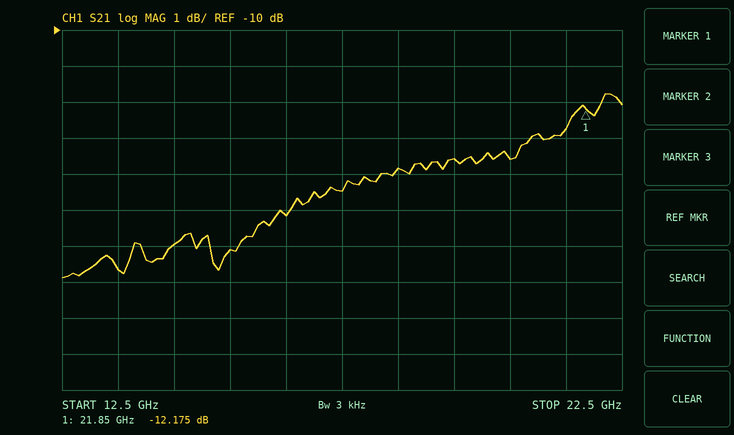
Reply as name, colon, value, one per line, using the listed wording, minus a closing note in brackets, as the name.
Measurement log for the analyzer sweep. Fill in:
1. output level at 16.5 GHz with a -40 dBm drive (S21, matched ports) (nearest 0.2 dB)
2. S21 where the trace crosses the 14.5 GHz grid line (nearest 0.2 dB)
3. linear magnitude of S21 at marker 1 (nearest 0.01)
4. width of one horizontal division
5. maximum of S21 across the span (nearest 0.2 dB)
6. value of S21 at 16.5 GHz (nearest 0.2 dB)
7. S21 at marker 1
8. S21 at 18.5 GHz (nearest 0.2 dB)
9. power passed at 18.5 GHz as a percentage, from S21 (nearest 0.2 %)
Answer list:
output level at 16.5 GHz with a -40 dBm drive (S21, matched ports): -55.2 dBm
S21 where the trace crosses the 14.5 GHz grid line: -16.0 dB
linear magnitude of S21 at marker 1: 0.25
width of one horizontal division: 1 GHz
maximum of S21 across the span: -11.8 dB
value of S21 at 16.5 GHz: -15.2 dB
S21 at marker 1: -12.175 dB
S21 at 18.5 GHz: -13.8 dB
power passed at 18.5 GHz as a percentage, from S21: 4.2 %
